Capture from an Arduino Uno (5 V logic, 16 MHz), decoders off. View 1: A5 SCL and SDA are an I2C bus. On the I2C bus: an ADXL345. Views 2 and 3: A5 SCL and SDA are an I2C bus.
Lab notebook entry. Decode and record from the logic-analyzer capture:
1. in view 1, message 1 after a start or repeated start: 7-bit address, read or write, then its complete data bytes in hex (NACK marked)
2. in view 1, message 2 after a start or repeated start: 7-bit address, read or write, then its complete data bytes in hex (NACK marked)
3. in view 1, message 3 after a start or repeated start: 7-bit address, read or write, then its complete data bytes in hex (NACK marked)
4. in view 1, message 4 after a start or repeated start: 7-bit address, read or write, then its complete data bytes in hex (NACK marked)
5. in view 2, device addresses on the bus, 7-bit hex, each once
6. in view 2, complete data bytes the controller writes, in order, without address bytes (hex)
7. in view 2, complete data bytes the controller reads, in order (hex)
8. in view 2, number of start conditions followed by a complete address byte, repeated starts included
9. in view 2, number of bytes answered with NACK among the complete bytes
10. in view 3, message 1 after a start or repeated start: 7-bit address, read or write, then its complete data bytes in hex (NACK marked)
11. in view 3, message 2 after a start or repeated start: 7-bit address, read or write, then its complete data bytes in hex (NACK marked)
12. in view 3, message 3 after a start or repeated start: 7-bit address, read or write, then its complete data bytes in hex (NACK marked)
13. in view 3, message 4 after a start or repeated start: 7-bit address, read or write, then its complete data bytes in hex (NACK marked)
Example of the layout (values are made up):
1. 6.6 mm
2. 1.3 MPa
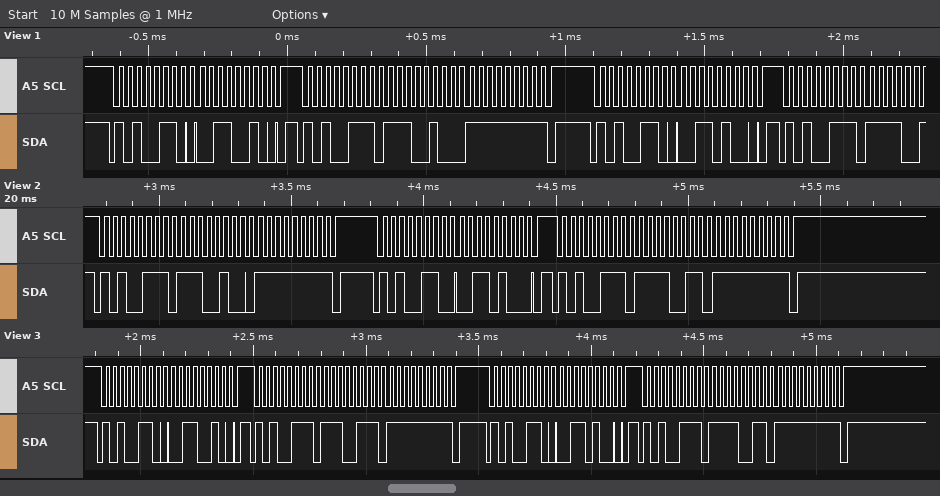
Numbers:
1. 0x53 write: 32
2. 0x53 read: E4 FF NACK
3. 0x53 write: 34
4. 0x53 read
5. 0x53
6. 34
7. E4 FF F3 FF
8. 3
9. 2
10. 0x53 write: 32
11. 0x53 read: E7 FF NACK
12. 0x53 write: 34
13. 0x53 read: F3 FF NACK
